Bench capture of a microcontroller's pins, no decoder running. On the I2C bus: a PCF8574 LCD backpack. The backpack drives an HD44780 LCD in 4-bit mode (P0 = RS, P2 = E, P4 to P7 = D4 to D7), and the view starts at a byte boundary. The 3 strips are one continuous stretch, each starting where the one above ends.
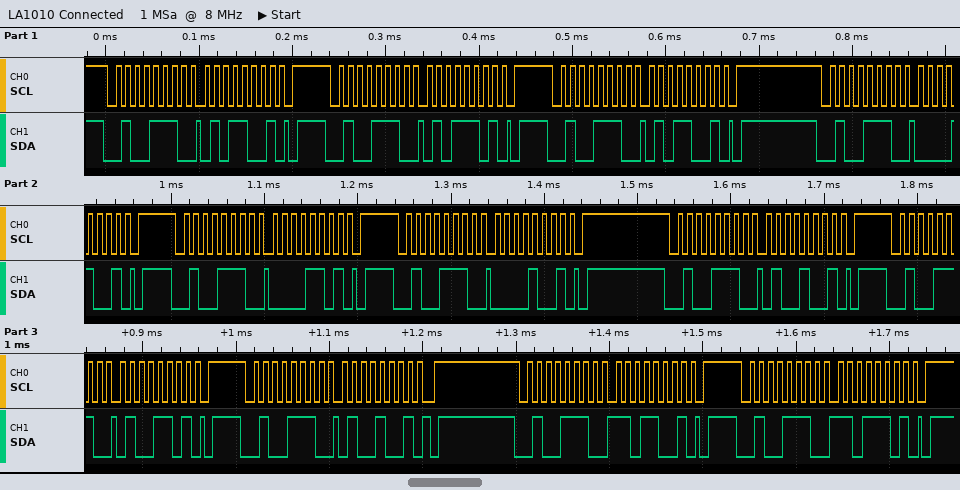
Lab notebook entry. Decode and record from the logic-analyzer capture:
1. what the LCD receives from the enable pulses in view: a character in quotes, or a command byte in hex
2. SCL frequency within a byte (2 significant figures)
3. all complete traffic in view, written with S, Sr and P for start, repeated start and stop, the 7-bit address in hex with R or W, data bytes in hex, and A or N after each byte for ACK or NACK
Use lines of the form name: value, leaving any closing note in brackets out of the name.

what the LCD receives from the enable pulses in view: a character in quotes, or a command byte in hex: 'P'
SCL frequency within a byte: 100 kHz
all complete traffic in view, written with S, Sr and P for start, repeated start and stop, the 7-bit address in hex with R or W, data bytes in hex, and A or N after each byte for ACK or NACK: S 27W A 59 A P S 27W A 5D A P S 27W A 59 A P S 27W A 09 A P S 27W A 0D A P S 27W A 09 A P S 27W A 49 A P S 27W A 4D A P S 27W A 49 A P S 27W A D9 A P S 27W A DD A P
